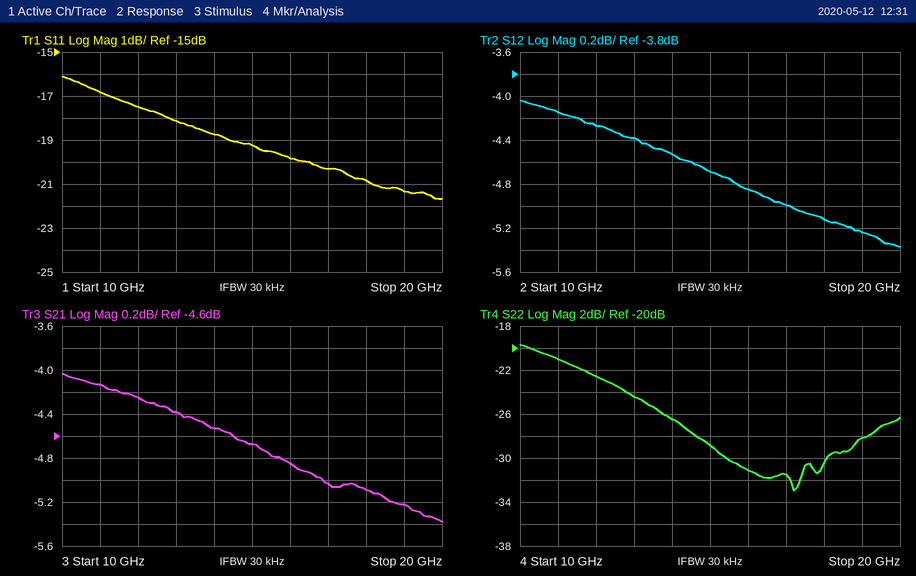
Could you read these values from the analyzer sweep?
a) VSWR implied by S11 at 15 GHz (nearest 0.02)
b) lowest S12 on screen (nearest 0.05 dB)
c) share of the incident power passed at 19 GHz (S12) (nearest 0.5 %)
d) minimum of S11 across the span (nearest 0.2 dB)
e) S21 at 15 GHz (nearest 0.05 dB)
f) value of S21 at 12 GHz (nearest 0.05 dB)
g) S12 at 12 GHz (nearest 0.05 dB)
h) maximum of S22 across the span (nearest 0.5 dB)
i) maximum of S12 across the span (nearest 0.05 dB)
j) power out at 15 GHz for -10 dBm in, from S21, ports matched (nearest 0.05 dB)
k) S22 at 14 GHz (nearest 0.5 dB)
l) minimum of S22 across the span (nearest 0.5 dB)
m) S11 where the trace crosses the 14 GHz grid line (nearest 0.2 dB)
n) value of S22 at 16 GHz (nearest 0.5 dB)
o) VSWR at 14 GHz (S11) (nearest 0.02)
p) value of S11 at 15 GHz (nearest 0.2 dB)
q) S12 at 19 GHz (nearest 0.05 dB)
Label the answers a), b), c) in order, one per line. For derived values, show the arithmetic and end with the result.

a) |Γ| = 10^(-19.2/20) = 0.1096; VSWR = (1 + 0.1096)/(1 − 0.1096) ≈ 1.25, so 1.24 to the nearest 0.02
b) -5.35 dB
c) 10^(-5.25/10) ≈ 29.9 %, so 30.0 % to the nearest 0.5 %
d) -21.6 dB
e) -4.65 dB
f) -4.25 dB
g) -4.25 dB
h) -19.5 dB
i) -4.05 dB
j) -10 dBm + (-4.65 dB) = -14.65 dBm
k) -26.5 dB
l) -33.0 dB
m) -18.8 dB
n) -31.0 dB
o) |Γ| = 10^(-18.8/20) = 0.1148; VSWR = (1 + 0.1148)/(1 − 0.1148) ≈ 1.26
p) -19.2 dB
q) -5.25 dB
